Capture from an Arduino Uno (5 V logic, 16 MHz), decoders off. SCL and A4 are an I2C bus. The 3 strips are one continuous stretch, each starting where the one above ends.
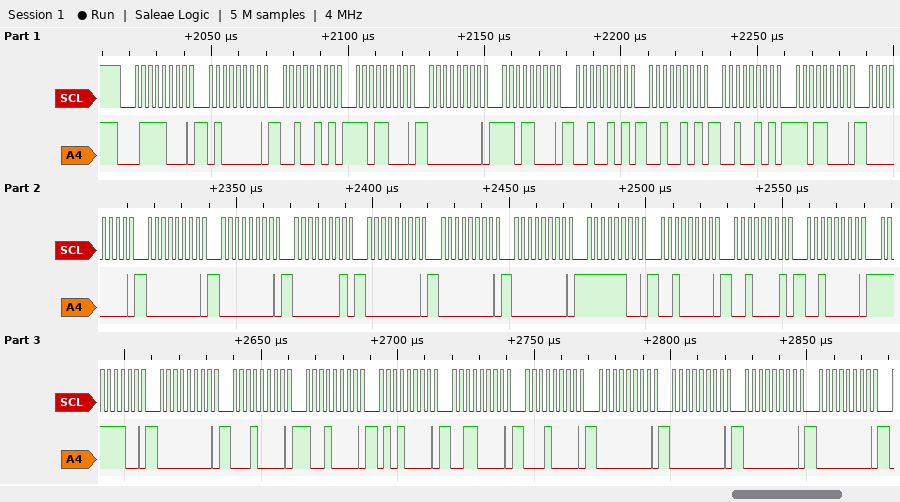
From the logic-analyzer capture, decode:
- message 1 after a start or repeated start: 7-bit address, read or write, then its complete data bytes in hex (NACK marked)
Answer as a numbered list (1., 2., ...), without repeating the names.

1. 0x3C write: 40 25 D8 00 D8 25 25 25 D8 00 00 00 01 00 00 00 FC 20 21 20 FC 00 10 90 50 30 10 00 00 00 00
